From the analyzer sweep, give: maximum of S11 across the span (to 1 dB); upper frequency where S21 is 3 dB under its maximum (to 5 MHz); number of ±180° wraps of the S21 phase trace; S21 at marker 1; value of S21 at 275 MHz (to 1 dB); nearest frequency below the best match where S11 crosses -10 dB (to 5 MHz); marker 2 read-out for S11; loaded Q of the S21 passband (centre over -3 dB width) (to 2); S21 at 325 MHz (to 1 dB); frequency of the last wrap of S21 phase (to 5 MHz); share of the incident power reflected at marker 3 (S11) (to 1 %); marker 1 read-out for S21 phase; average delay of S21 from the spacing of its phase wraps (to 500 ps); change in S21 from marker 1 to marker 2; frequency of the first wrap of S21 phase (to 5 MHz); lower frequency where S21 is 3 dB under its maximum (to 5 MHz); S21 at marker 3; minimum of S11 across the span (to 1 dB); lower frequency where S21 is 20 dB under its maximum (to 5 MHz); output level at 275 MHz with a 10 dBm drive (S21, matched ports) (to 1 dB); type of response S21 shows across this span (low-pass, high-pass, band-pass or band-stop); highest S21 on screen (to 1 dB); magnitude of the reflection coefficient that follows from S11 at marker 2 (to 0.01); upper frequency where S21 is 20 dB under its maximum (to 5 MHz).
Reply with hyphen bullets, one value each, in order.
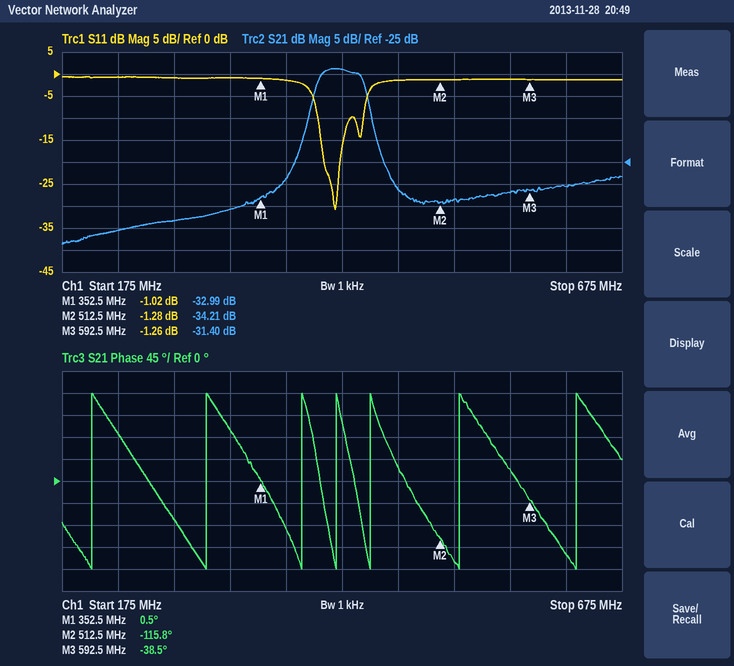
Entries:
- -1 dB
- 445 MHz
- 7
- -32.99 dB
- -38 dB
- 405 MHz
- -1.28 dB
- 10
- -36 dB
- 635 MHz
- 75 %
- 0.5°
- 14.0 ns
- -1.22 dB
- 200 MHz
- 405 MHz
- -31.40 dB
- -31 dB
- 385 MHz
- -28 dBm
- band-pass
- -4 dB
- 0.86
- 460 MHz
